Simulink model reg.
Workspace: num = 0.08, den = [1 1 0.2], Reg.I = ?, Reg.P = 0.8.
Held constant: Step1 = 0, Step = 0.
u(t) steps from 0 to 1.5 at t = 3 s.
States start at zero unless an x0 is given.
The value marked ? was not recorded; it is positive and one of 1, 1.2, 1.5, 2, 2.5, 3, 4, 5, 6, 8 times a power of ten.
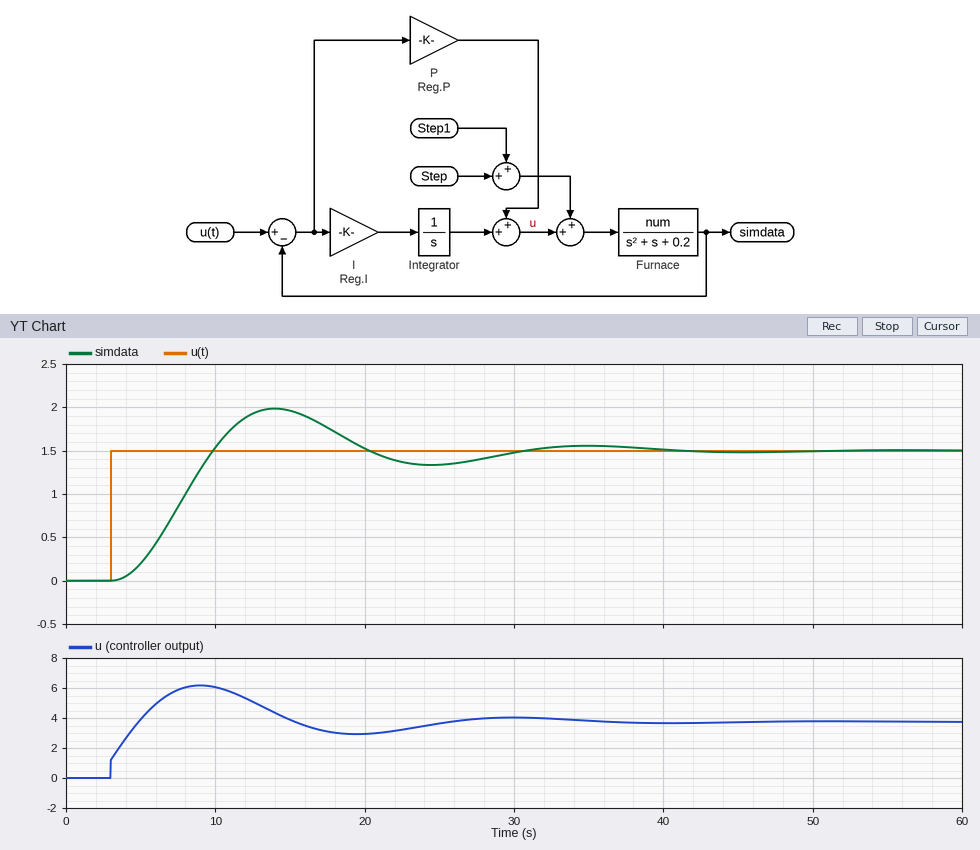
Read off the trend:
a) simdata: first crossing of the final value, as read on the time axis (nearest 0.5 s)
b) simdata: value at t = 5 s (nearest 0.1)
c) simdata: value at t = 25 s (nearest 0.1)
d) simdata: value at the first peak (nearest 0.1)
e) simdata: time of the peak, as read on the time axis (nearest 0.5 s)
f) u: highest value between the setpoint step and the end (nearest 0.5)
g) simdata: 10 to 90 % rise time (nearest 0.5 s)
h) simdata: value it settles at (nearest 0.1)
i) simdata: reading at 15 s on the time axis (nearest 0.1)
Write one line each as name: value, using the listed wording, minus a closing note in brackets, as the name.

simdata: first crossing of the final value, as read on the time axis: 10.0 s
simdata: value at t = 5 s: 0.2
simdata: value at t = 25 s: 1.3
simdata: value at the first peak: 2.0
simdata: time of the peak, as read on the time axis: 14.0 s
u: highest value between the setpoint step and the end: 6.0
simdata: 10 to 90 % rise time: 4.5 s
simdata: value it settles at: 1.5
simdata: reading at 15 s on the time axis: 2.0
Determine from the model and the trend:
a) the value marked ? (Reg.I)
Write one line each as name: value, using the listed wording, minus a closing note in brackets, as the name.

the value marked ?: 1
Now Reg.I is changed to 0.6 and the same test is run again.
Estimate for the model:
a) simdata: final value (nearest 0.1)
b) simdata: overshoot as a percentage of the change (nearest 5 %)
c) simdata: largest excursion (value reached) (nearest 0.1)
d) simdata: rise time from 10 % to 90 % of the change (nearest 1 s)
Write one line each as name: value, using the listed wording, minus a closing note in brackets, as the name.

simdata: final value: 1.5
simdata: overshoot as a percentage of the change: 15 %
simdata: largest excursion (value reached): 1.7
simdata: rise time from 10 % to 90 % of the change: 7 s
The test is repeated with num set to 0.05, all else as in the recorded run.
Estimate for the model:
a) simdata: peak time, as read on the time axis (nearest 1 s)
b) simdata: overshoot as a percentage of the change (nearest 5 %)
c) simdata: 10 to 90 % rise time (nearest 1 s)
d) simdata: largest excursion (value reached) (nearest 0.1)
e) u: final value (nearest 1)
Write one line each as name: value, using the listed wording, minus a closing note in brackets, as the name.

simdata: peak time, as read on the time axis: 17 s
simdata: overshoot as a percentage of the change: 20 %
simdata: 10 to 90 % rise time: 6 s
simdata: largest excursion (value reached): 1.8
u: final value: 6
